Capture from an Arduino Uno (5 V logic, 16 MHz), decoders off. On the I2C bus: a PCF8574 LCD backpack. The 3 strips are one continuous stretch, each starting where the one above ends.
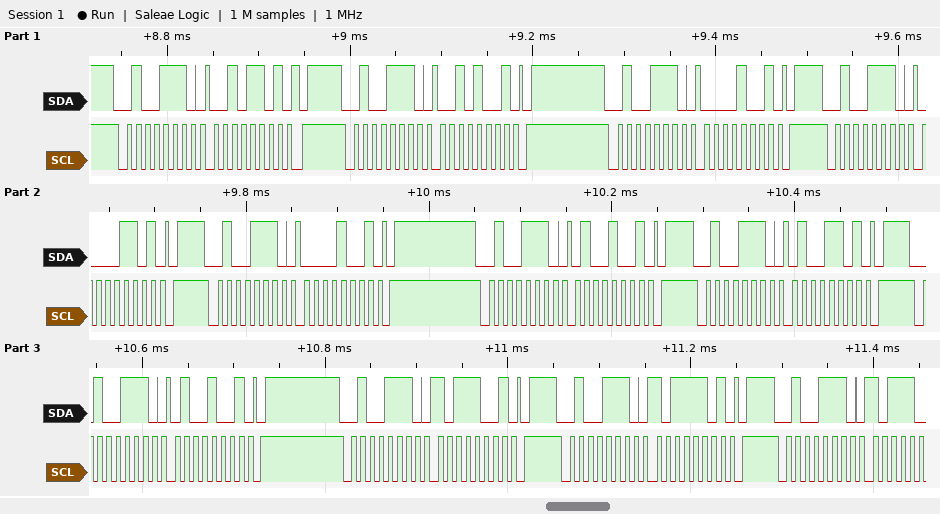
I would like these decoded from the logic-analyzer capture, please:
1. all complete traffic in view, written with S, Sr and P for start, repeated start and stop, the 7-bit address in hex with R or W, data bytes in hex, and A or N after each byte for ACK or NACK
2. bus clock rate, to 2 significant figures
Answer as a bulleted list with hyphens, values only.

- S 27W A 2D A P S 27W A 29 A P S 27W A 09 A P S 27W A 0D A P S 27W A 09 A P S 27W A 49 A P S 27W A 4D A P S 27W A 49 A P S 27W A B9 A P S 27W A BD A P S 27W A
- 100 kHz
